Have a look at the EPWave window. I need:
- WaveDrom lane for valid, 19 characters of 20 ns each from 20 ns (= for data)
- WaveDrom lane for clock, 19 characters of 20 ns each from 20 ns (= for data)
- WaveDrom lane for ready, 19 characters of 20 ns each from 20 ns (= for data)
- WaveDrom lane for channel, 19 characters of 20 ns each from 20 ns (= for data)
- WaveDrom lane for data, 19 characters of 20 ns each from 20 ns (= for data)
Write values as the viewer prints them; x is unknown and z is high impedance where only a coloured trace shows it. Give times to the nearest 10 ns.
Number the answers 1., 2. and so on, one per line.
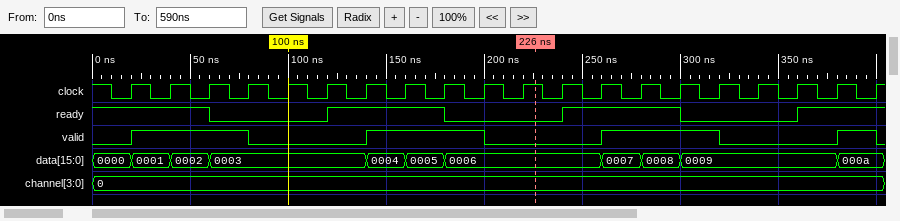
1. {name: 'valid', wave: '1..0..1..0..1..0..1'}
2. {name: 'clock', wave: 'p..................'}
3. {name: 'ready', wave: '1.0..1..0..1..0..1.'}
4. {name: 'channel', wave: '=..................', data: '0'}
5. {name: 'data', wave: '===...===...===...=', data: '0001 0002 0003 0004 0005 0006 0007 0008 0009 000a'}
